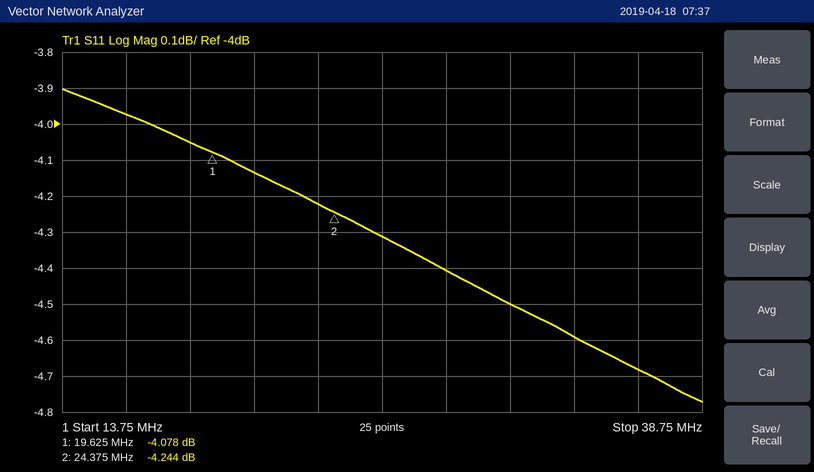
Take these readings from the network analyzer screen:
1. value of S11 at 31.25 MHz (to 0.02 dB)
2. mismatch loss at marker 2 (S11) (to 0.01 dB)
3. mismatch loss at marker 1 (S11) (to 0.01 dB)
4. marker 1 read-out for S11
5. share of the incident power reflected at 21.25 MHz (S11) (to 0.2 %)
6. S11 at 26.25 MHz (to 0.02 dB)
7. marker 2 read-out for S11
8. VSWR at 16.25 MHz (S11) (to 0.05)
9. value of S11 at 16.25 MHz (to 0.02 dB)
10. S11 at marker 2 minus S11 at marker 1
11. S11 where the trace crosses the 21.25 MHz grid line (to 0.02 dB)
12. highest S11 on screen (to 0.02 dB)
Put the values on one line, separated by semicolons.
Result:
-4.50 dB; 2.05 dB; 2.15 dB; -4.078 dB; 38.6 %; -4.32 dB; -4.244 dB; 4.45; -3.98 dB; -0.166 dB; -4.14 dB; -3.90 dB
